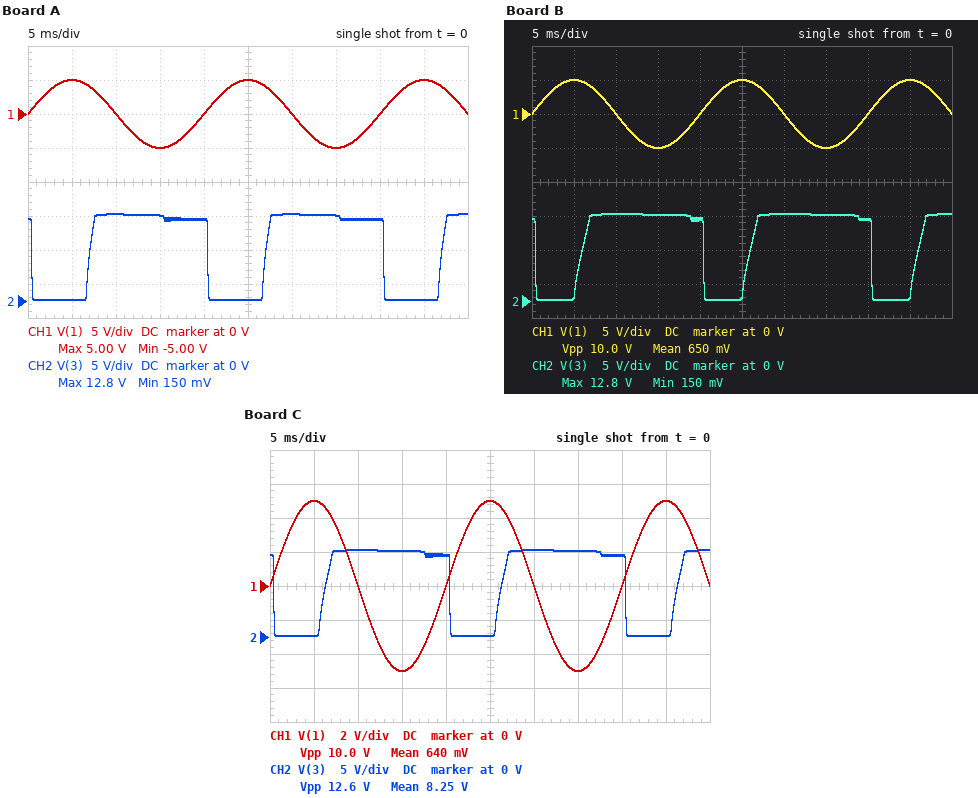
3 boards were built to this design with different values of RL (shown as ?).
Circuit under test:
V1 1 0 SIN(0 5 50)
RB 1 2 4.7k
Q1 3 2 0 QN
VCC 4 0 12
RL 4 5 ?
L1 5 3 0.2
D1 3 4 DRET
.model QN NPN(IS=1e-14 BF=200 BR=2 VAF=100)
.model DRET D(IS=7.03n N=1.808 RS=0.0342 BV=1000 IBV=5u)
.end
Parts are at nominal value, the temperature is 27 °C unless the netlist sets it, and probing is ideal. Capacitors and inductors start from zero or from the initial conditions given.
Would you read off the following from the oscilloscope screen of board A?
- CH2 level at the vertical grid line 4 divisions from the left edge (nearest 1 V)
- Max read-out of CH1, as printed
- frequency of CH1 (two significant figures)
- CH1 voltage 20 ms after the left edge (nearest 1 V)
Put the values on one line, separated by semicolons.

12 V; 5.00 V; 50 Hz; 0 V
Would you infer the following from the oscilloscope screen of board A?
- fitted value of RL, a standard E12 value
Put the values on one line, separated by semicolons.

68 Ω
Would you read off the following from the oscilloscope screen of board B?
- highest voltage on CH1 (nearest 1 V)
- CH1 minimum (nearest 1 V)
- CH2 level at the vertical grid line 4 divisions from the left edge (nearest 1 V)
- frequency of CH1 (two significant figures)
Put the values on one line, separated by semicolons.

5 V; -5 V; 12 V; 50 Hz
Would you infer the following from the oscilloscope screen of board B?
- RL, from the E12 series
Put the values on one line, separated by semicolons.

39 Ω
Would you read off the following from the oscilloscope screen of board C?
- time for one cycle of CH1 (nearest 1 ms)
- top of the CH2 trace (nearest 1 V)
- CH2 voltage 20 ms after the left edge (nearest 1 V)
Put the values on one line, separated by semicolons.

20 ms; 13 V; 12 V
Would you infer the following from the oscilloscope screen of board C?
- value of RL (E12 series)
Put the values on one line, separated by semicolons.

47 Ω
